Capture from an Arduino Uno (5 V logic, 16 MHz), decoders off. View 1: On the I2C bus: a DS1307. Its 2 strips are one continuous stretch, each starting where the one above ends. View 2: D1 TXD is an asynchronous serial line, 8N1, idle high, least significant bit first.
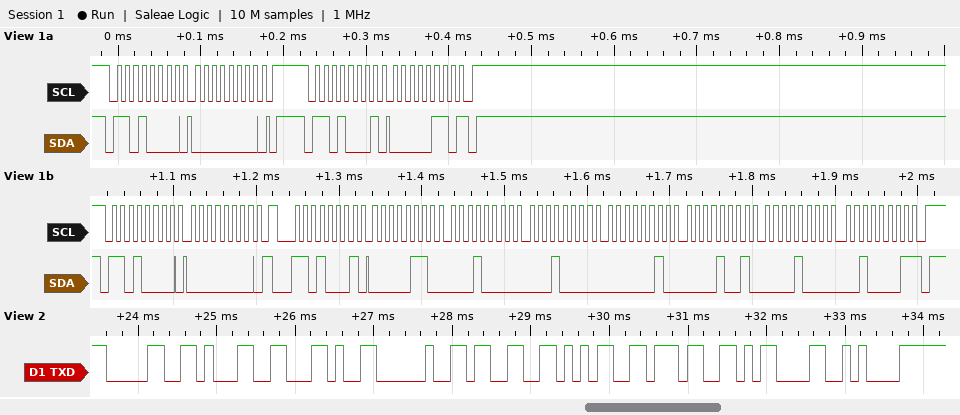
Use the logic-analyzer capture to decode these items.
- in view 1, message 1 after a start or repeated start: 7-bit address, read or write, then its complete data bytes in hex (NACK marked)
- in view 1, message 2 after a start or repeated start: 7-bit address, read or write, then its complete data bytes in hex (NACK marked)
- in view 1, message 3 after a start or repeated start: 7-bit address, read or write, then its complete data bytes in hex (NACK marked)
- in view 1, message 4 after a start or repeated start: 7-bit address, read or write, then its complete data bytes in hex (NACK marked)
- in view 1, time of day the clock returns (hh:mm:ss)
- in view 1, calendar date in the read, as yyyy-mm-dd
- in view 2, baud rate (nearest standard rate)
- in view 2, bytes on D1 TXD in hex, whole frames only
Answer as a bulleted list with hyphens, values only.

- 0x68 write: 00
- 0x68 read: 06 NACK
- 0x68 write: 00
- 0x68 read: 06 10 10 02 09 08 21 NACK
- 10:10:06
- 2021-08-09
- 9600 baud
- 30 31 2C 20 33 35 37 0D 0A
